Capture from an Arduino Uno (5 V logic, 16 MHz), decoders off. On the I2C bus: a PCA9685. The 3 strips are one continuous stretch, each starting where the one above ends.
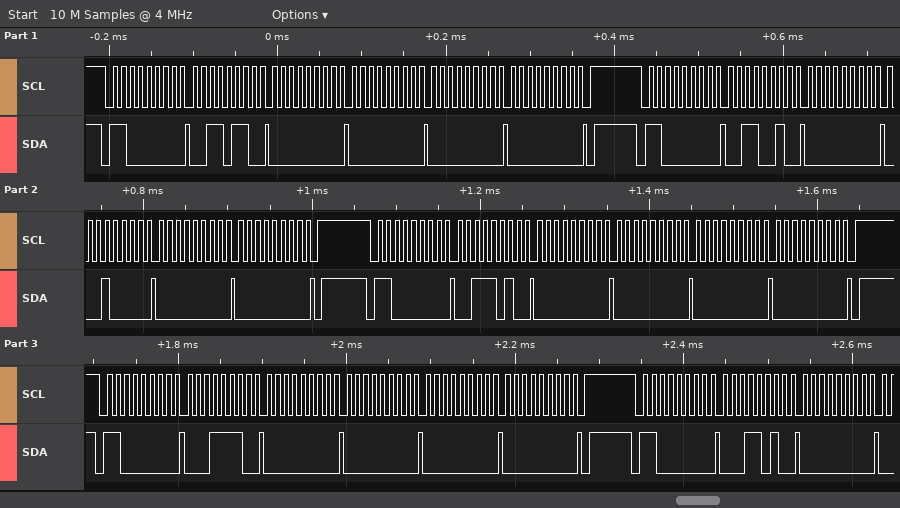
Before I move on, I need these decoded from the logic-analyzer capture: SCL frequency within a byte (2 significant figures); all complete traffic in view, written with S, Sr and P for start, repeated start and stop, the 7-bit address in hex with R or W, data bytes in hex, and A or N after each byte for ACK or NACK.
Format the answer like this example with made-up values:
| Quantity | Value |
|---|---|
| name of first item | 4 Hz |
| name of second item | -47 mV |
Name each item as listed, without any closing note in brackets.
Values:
| Quantity | Value |
|---|---|
| SCL frequency within a byte | 100 kHz |
| all complete traffic in view, written with S, Sr and P for start, repeated start and stop, the 7-bit address in hex with R or W, data bytes in hex, and A or N after each byte for ACK or NACK | S 60W A 36 A 00 A 00 A 00 A 00 A P S 60W A 32 A 00 A 10 A 00 A 00 A P S 60W A 3A A 00 A 00 A 00 A 00 A P S 60W A 1E A 00 A 00 A 00 A 00 A P S 60W A 1A A 00 A |
